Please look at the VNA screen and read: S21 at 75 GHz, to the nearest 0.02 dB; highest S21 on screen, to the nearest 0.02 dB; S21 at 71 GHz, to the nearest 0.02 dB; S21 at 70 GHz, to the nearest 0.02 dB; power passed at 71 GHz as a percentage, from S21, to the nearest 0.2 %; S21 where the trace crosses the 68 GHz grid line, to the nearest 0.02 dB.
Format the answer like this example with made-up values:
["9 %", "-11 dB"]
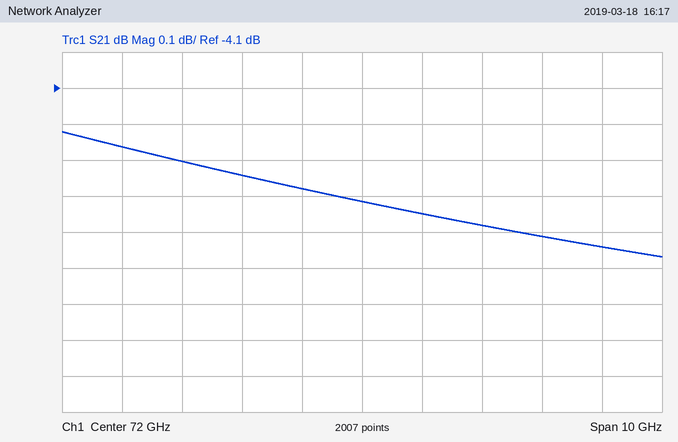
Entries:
["-4.52 dB", "-4.22 dB", "-4.38 dB", "-4.34 dB", "36.4 %", "-4.26 dB"]
